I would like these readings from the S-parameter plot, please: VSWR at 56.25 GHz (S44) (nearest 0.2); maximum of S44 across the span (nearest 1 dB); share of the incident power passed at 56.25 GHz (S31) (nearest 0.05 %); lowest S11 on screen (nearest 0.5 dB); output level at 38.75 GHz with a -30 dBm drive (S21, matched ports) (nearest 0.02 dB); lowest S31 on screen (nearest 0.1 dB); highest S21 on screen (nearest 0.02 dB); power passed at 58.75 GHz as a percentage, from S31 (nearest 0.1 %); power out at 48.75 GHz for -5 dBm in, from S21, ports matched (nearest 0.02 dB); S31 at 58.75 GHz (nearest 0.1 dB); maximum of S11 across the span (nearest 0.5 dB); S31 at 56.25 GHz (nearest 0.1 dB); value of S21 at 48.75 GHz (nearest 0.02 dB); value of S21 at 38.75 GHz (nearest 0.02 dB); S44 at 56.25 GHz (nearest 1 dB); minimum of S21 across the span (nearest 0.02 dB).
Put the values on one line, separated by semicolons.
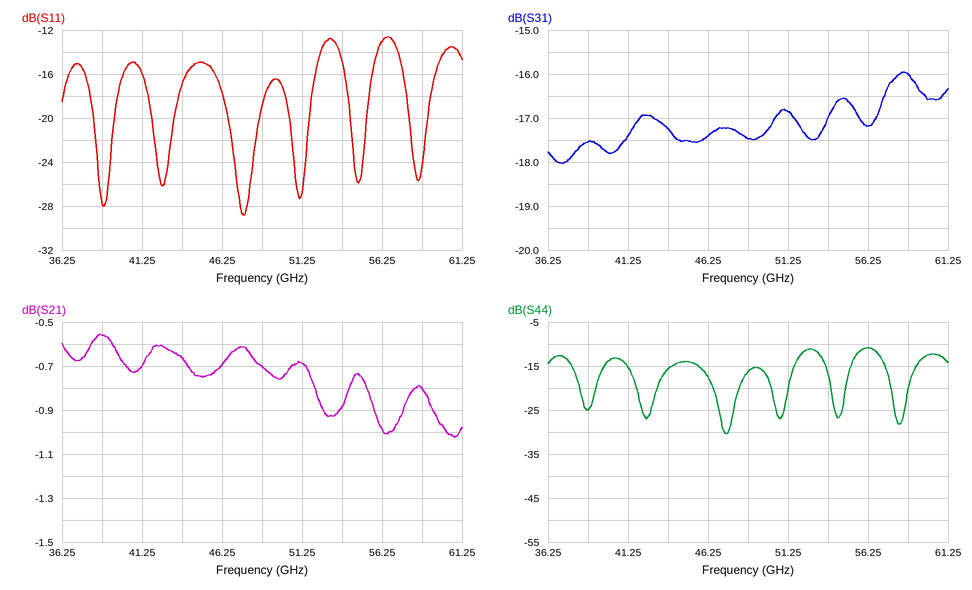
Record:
1.8; -11 dB; 1.90 %; -29.0 dB; -30.56 dBm; -18.0 dB; -0.56 dB; 2.5 %; -5.70 dBm; -16.0 dB; -12.5 dB; -17.2 dB; -0.70 dB; -0.56 dB; -11 dB; -1.02 dB
